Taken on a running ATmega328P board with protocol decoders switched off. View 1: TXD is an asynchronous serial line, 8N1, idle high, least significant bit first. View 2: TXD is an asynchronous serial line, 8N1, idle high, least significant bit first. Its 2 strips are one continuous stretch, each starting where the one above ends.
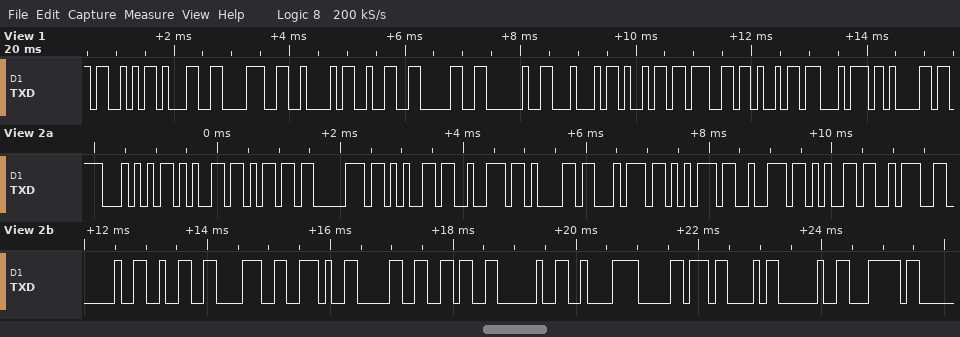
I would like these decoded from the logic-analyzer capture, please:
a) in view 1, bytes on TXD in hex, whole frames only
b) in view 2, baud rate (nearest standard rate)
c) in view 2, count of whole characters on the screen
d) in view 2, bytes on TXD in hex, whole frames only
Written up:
53 31 38 42 32 30 20 44 69 67 69 74 61
9600 baud
24
0x54 0x65 0x6D 0x70 0x65 0x72 0x61 0x74 0x75 0x72 0x65 0x3A 0x20 0x32 0x38 0x2E 0x30 0x36 0x20 0xC2 0xB0 0x43 0x20 0x7C
